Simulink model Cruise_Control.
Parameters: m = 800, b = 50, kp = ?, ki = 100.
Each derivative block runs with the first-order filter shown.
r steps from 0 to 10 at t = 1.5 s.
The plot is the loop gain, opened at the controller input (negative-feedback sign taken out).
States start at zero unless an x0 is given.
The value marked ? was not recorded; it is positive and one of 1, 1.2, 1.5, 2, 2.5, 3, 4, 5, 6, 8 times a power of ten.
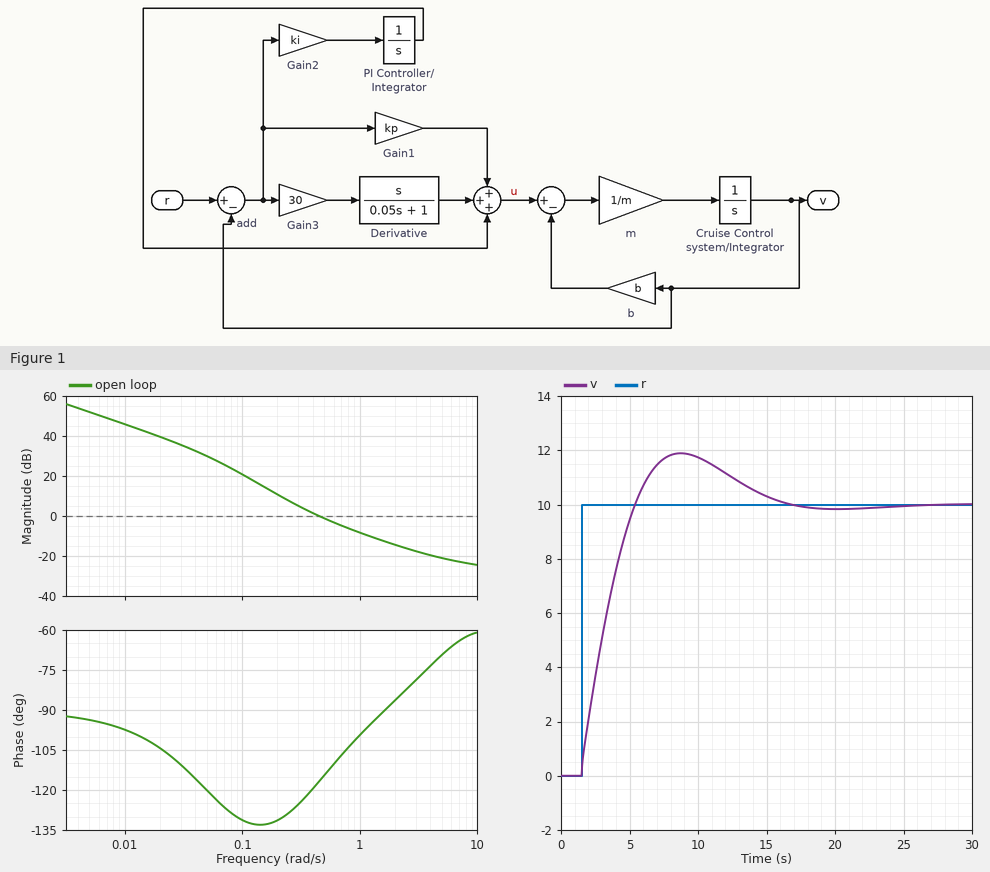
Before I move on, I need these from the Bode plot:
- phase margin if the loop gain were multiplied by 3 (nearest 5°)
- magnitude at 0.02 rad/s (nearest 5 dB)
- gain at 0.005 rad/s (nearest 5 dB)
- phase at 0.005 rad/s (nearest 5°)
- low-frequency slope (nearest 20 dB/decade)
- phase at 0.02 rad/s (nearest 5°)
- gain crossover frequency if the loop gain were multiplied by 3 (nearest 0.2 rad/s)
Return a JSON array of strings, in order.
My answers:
["85°", "40 dB", "50 dB", "-95°", "-20 dB/decade", "-105°", "1.2 rad/s"]
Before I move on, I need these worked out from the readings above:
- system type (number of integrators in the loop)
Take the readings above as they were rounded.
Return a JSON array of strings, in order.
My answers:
["1"]
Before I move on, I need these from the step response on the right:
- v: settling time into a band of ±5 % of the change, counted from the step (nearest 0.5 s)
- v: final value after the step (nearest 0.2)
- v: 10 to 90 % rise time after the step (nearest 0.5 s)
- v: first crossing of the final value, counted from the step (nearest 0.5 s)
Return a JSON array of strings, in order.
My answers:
["12.5 s", "10.0", "3.0 s", "4.0 s"]
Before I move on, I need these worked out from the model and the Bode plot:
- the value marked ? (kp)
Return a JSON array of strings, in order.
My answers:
["300"]
